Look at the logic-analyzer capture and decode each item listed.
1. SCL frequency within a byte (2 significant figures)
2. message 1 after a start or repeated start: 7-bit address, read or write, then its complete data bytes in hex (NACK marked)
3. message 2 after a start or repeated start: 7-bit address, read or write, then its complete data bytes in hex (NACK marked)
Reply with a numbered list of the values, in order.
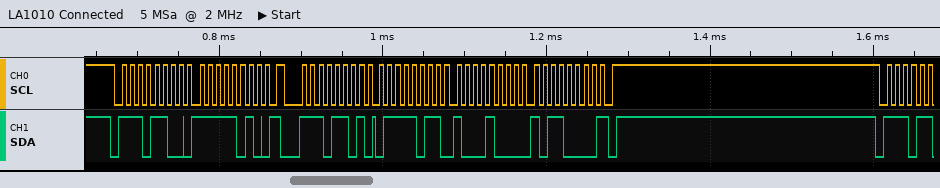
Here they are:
1. 100 kHz
2. 0x76 write: FA
3. 0x76 read: 7B 88 B0 NACK
